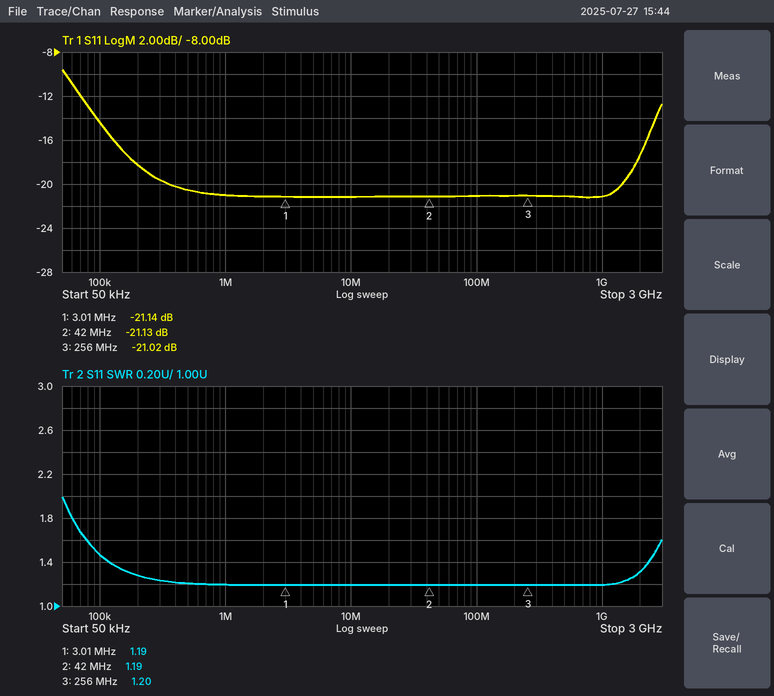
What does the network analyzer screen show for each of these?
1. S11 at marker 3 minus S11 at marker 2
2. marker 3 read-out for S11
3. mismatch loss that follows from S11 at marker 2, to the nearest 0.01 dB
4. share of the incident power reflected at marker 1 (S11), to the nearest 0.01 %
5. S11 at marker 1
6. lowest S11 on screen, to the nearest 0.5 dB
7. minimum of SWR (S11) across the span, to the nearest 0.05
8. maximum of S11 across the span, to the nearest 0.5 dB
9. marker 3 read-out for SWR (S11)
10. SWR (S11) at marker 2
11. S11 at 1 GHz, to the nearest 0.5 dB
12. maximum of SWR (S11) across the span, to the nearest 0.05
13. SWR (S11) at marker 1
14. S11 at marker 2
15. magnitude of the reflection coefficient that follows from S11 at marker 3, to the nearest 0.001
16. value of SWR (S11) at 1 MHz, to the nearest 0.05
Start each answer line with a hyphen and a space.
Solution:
- 0.11 dB
- -21.02 dB
- 0.03 dB
- 0.77 %
- -21.14 dB
- -21.0 dB
- 1.20
- -9.5 dB
- 1.20
- 1.19
- -21.0 dB
- 2.00
- 1.19
- -21.13 dB
- 0.089
- 1.20
